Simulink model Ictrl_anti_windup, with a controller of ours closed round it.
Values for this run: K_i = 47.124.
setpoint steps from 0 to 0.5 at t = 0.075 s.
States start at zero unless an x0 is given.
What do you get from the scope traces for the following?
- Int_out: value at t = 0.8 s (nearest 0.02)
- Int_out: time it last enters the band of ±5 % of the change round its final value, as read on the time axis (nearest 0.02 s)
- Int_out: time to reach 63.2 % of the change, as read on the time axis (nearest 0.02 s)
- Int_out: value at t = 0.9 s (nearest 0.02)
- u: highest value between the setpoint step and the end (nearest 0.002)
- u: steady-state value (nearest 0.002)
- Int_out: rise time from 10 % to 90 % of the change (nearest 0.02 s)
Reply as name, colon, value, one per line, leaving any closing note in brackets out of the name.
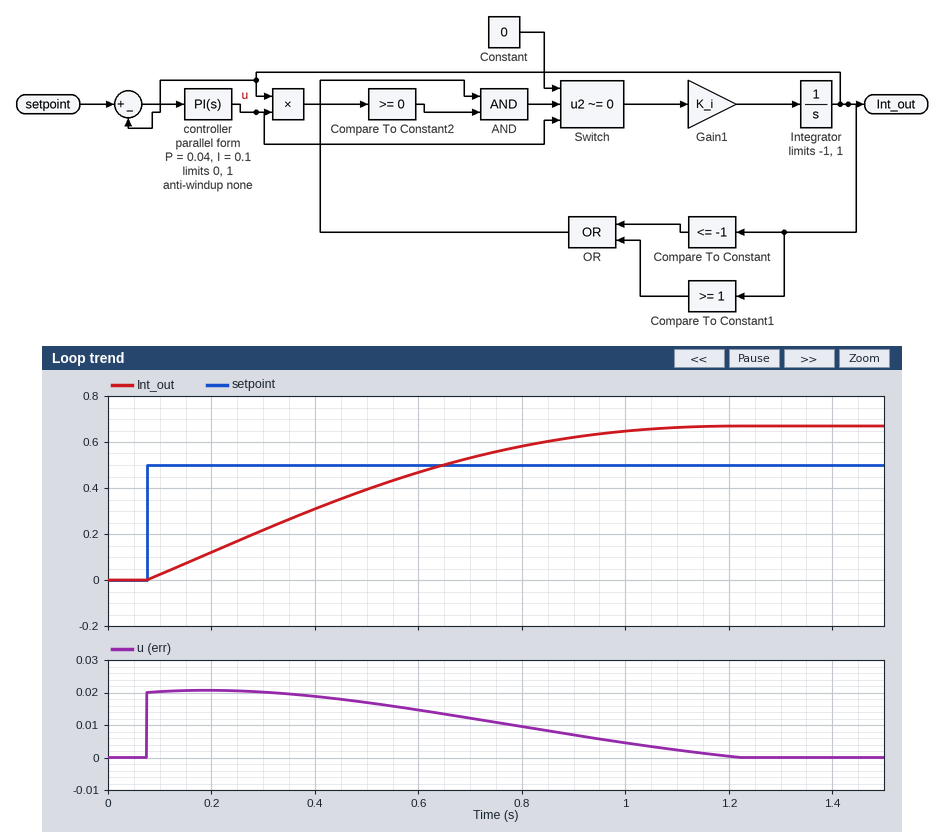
Int_out: value at t = 0.8 s: 0.58
Int_out: time it last enters the band of ±5 % of the change round its final value, as read on the time axis: 0.96 s
Int_out: time to reach 63.2 % of the change, as read on the time axis: 0.54 s
Int_out: value at t = 0.9 s: 0.62
u: highest value between the setpoint step and the end: 0.020
u: steady-state value: 0.000
Int_out: rise time from 10 % to 90 % of the change: 0.70 s
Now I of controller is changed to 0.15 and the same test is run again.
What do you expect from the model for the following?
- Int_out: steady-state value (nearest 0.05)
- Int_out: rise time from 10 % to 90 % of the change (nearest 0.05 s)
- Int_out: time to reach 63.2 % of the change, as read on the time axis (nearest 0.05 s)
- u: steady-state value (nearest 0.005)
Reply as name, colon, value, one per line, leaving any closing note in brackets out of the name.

Int_out: steady-state value: 0.70
Int_out: rise time from 10 % to 90 % of the change: 0.60 s
Int_out: time to reach 63.2 % of the change, as read on the time axis: 0.50 s
u: steady-state value: 0.000
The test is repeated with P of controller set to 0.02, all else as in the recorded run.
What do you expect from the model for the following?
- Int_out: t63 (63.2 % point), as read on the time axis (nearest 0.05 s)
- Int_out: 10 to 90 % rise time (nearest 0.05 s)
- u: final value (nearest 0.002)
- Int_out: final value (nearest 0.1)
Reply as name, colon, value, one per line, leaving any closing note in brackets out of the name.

Int_out: t63 (63.2 % point), as read on the time axis: 0.70 s
Int_out: 10 to 90 % rise time: 0.80 s
u: final value: 0.000
Int_out: final value: 0.8
